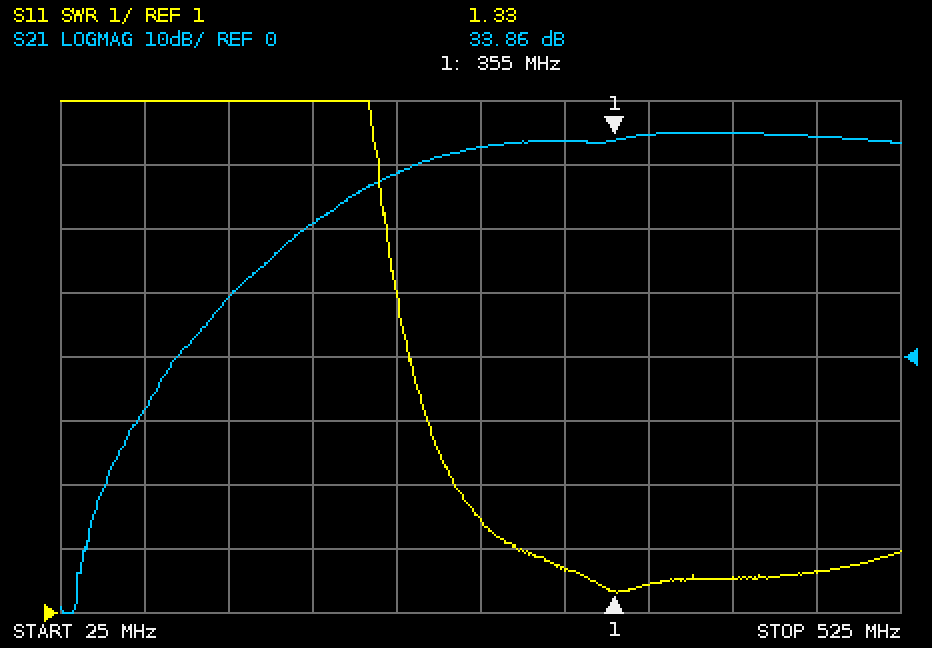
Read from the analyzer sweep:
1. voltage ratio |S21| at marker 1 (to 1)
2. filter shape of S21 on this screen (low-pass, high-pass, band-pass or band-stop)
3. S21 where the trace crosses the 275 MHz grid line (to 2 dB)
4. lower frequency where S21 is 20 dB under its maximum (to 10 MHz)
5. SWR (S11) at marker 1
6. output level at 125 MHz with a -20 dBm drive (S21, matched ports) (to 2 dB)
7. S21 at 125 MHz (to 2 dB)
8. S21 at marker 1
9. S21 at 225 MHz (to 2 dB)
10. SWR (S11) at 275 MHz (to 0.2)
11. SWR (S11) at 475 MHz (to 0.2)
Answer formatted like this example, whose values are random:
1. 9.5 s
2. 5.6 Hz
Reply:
1. 49
2. high-pass
3. 32 dB
4. 150 MHz
5. 1.33
6. -10 dBm
7. 10 dB
8. 33.86 dB
9. 28 dB
10. 2.4
11. 1.6
